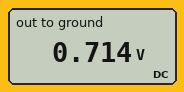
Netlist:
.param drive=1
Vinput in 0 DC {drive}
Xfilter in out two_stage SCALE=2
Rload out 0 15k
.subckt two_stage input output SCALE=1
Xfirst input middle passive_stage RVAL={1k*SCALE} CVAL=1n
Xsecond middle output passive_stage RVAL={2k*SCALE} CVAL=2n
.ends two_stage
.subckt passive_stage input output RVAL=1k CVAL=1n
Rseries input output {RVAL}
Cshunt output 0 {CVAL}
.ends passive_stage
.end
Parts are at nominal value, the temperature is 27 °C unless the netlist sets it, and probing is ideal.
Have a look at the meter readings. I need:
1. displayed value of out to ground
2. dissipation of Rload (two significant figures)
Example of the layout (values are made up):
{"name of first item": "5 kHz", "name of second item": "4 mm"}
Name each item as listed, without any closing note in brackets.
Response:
{"displayed value of out to ground": "0.714 V", "dissipation of Rload": "34 µW"}
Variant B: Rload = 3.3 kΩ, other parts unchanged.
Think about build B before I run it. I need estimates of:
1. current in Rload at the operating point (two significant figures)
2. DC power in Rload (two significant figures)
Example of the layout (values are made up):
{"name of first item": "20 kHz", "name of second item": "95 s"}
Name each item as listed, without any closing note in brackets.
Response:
{"current in Rload at the operating point": "110 µA", "DC power in Rload": "38 µW"}
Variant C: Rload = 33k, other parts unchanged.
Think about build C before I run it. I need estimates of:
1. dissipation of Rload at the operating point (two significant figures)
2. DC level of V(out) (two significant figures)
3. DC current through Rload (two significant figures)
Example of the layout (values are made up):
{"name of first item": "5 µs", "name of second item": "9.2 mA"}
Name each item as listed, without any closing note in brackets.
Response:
{"dissipation of Rload at the operating point": "22 µW", "DC level of V(out)": "850 mV", "DC current through Rload": "26 µA"}
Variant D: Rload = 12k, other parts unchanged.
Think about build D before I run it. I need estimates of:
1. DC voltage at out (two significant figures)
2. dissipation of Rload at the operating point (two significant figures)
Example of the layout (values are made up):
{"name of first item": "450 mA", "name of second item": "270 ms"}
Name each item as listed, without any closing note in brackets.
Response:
{"DC voltage at out": "670 mV", "dissipation of Rload at the operating point": "37 µW"}
